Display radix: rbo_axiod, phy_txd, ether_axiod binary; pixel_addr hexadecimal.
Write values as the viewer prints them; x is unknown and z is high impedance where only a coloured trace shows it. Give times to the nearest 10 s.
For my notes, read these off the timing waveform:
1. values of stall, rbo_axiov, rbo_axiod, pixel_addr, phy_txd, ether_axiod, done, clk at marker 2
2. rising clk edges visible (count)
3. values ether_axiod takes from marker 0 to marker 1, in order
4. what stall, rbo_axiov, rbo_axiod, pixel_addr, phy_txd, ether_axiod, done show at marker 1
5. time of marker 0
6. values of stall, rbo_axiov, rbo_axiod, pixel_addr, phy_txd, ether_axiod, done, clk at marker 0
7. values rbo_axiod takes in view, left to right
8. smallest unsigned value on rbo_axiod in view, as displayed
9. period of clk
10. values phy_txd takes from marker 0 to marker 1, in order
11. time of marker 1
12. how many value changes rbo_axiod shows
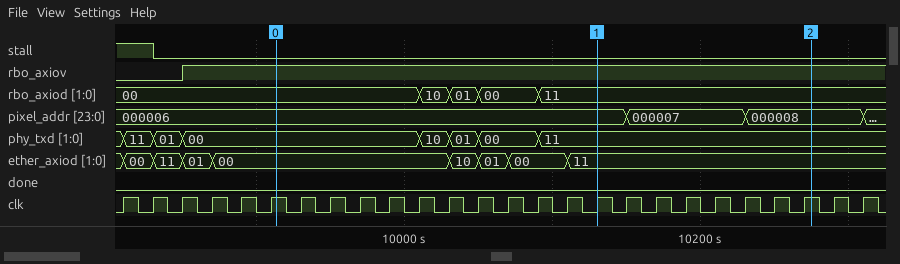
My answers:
stall=0, rbo_axiov=1, rbo_axiod=11, pixel_addr=000008, phy_txd=11, ether_axiod=11, done=0, clk=1
26
00, 10, 01, 00, 11
stall=0, rbo_axiov=1, rbo_axiod=11, pixel_addr=000006, phy_txd=11, ether_axiod=11, done=0
9910 s
stall=0, rbo_axiov=1, rbo_axiod=00, pixel_addr=000006, phy_txd=00, ether_axiod=00, done=0, clk=1
00, 10, 01, 00, 11
00
20 s
00, 10, 01, 00, 11
10130 s
4
